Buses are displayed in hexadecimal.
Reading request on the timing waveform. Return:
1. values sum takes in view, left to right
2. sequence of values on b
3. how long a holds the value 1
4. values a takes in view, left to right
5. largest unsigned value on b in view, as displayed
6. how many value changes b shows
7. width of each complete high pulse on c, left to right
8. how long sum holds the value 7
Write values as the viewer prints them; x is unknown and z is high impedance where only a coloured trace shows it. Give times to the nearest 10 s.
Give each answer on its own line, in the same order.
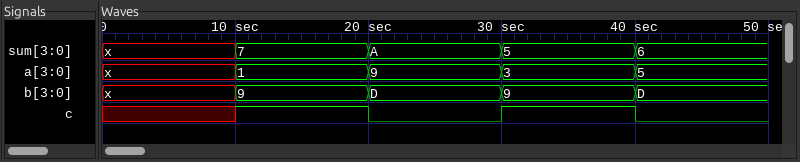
x, 7, A, 5, 6
x, 9, D, 9, D
10 s
x, 1, 9, 3, 5
D
4
10 s
10 s
